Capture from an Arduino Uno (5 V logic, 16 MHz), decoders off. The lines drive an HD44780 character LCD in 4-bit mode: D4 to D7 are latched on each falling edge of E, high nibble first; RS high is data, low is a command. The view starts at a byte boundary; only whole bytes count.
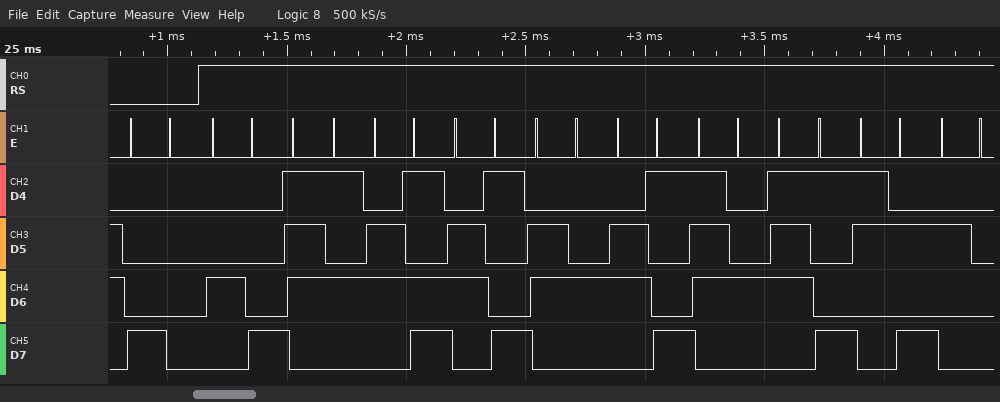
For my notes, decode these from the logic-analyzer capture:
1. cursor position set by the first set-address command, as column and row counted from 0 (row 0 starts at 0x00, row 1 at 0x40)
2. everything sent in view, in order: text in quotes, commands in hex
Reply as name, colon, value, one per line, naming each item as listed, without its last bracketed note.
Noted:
cursor position set by the first set-address command, as column and row counted from 0: column 0, row 0
everything sent in view, in order: text in quotes, commands in hex: 0x80 "Humidity: "
